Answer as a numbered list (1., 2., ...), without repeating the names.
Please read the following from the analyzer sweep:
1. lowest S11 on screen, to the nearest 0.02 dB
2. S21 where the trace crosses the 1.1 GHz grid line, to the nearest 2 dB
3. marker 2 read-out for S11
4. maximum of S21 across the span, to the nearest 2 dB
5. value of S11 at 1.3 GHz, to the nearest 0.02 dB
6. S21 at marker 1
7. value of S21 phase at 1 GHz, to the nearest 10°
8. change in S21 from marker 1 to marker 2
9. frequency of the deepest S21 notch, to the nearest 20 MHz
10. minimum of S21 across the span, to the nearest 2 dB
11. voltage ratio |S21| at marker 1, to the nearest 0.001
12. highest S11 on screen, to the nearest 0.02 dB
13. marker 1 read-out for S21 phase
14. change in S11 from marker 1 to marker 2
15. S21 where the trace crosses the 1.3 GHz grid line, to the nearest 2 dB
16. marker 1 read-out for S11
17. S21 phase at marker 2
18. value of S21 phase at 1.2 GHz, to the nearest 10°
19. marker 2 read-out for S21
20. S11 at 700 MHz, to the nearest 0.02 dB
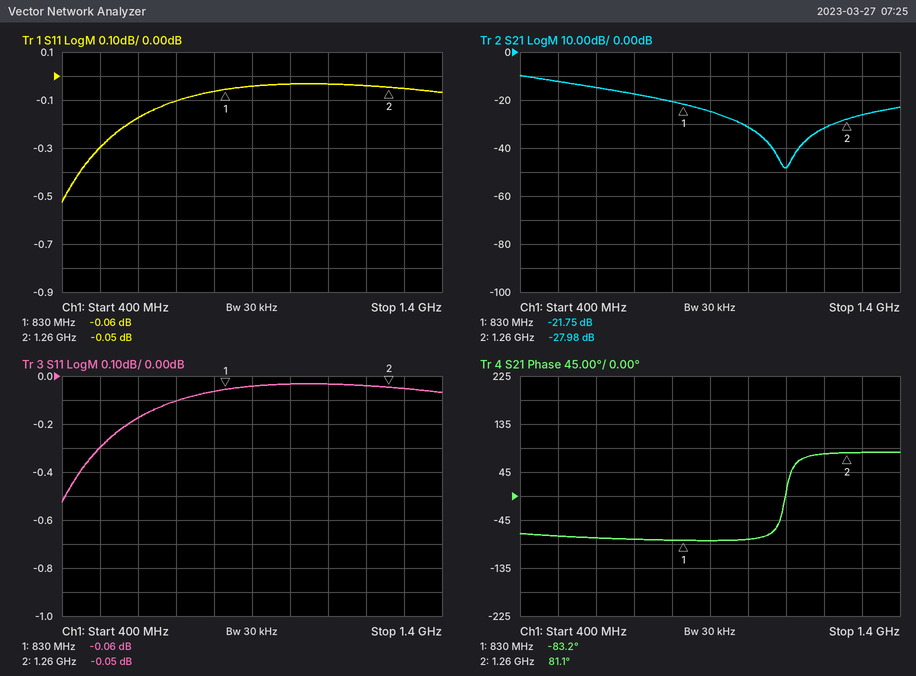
1. -0.52 dB
2. -48 dB
3. -0.05 dB
4. -10 dB
5. -0.06 dB
6. -21.75 dB
7. -80°
8. -6.23 dB
9. 1.10 GHz
10. -48 dB
11. 0.082
12. -0.04 dB
13. -83.2°
14. 0.01 dB
15. -26 dB
16. -0.06 dB
17. 81.1°
18. 80°
19. -27.98 dB
20. -0.10 dB
